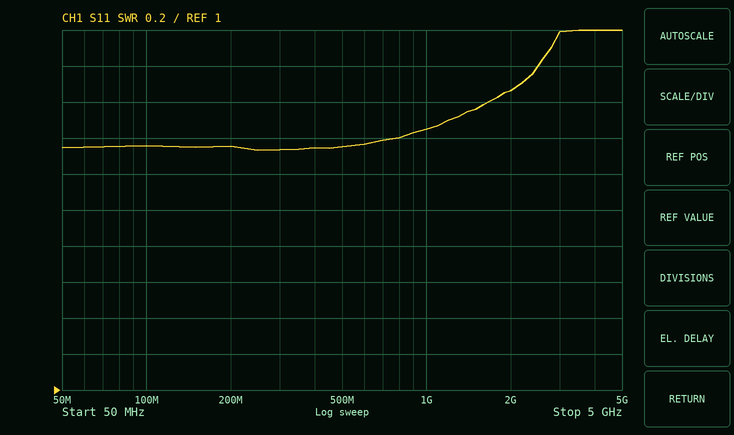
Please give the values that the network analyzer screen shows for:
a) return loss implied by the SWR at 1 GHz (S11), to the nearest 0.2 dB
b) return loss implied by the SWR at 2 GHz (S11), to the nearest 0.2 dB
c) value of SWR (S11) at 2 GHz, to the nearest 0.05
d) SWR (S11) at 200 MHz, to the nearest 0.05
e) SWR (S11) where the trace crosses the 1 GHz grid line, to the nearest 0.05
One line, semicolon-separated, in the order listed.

7.6 dB; 6.8 dB; 2.65; 2.35; 2.45
